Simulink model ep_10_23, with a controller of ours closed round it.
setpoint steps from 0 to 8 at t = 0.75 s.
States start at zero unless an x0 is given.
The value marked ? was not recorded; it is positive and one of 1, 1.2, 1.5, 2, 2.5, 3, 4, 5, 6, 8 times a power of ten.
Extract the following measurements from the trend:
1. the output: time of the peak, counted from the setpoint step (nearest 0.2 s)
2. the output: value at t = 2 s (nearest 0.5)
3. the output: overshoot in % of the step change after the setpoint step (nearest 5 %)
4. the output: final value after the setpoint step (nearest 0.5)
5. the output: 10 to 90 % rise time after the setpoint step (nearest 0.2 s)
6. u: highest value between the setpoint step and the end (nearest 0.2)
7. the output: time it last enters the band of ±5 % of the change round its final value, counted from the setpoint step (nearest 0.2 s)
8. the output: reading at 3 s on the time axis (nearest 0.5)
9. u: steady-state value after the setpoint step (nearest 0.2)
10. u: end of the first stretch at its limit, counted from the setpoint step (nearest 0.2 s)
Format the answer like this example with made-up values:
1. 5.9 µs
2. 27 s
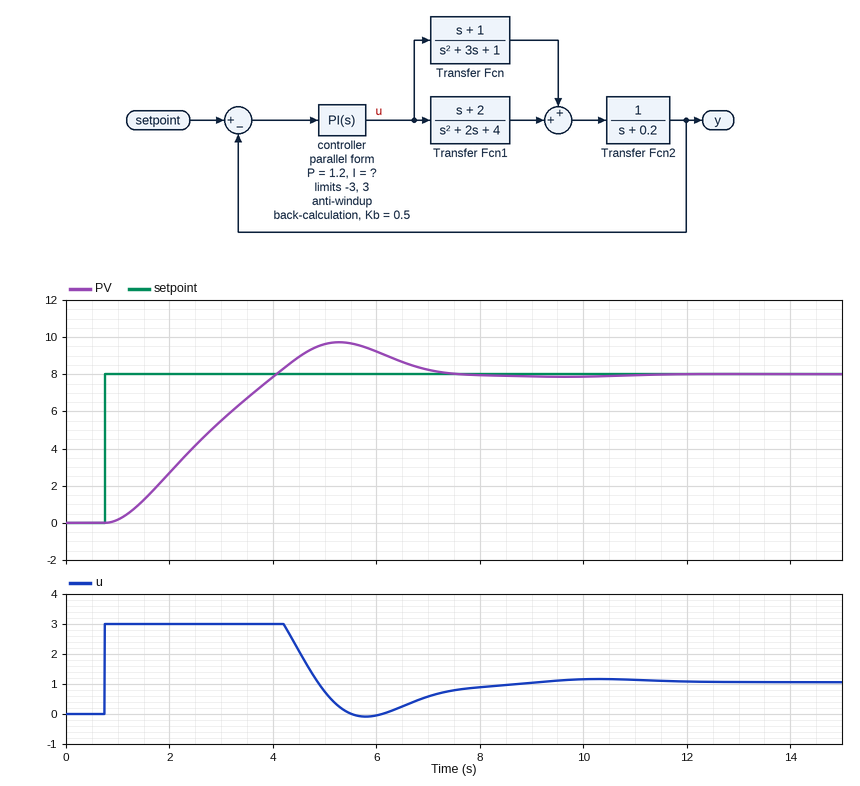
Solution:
1. 4.6 s
2. 2.5
3. 20 %
4. 8.0
5. 2.4 s
6. 3.0
7. 6.0 s
8. 5.5
9. 1.0
10. 3.4 s
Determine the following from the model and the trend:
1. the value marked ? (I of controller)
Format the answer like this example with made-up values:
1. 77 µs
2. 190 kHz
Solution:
1. 0.8
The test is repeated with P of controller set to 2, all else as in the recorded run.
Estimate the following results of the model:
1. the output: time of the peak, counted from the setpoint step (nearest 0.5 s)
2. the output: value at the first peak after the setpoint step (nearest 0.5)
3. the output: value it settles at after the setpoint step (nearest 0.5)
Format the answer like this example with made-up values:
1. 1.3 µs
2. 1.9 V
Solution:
1. 4.0 s
2. 8.5
3. 8.0
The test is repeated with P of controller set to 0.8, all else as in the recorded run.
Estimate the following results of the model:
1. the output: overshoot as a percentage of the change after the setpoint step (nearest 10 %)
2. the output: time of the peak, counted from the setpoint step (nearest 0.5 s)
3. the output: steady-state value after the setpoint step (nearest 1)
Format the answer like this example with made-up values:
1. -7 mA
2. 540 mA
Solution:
1. 30 %
2. 5.0 s
3. 8
